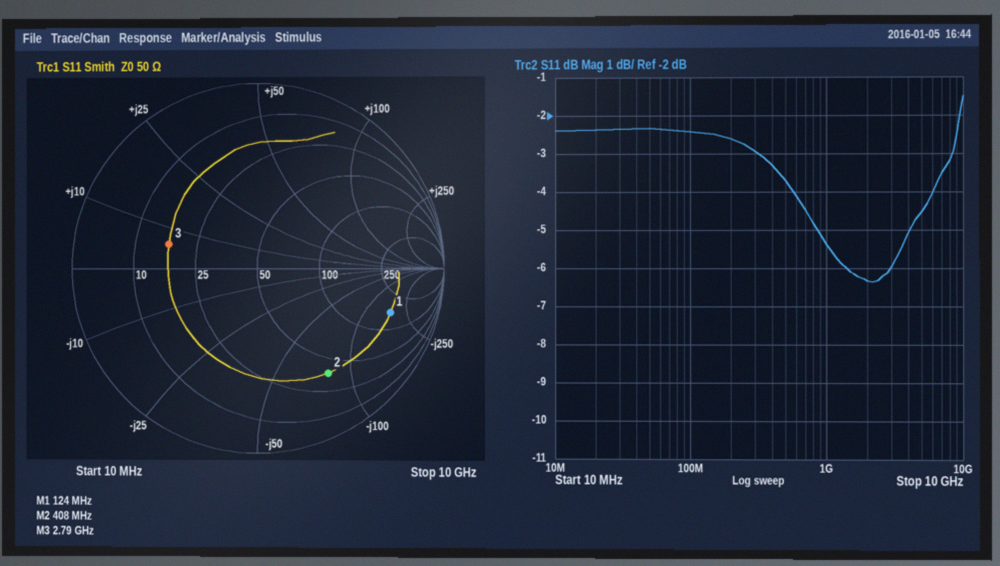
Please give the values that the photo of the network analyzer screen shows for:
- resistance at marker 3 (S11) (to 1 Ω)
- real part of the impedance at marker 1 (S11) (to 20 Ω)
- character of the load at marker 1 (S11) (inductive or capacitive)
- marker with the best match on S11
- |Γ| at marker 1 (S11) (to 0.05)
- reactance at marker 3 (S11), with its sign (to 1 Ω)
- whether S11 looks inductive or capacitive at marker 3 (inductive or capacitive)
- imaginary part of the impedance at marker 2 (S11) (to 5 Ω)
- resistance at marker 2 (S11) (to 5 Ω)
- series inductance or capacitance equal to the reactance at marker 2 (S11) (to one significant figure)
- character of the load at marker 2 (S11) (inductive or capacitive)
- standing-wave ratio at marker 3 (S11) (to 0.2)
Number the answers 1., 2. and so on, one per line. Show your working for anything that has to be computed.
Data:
1. 17 Ω
2. 160 Ω
3. capacitive
4. marker 3
5. 0.75
6. +6 Ω
7. inductive
8. -80 Ω
9. 40 Ω
10. C = 1/(2π × 408 MHz × 80 Ω) ≈ 5 pF
11. capacitive
12. 3.0
